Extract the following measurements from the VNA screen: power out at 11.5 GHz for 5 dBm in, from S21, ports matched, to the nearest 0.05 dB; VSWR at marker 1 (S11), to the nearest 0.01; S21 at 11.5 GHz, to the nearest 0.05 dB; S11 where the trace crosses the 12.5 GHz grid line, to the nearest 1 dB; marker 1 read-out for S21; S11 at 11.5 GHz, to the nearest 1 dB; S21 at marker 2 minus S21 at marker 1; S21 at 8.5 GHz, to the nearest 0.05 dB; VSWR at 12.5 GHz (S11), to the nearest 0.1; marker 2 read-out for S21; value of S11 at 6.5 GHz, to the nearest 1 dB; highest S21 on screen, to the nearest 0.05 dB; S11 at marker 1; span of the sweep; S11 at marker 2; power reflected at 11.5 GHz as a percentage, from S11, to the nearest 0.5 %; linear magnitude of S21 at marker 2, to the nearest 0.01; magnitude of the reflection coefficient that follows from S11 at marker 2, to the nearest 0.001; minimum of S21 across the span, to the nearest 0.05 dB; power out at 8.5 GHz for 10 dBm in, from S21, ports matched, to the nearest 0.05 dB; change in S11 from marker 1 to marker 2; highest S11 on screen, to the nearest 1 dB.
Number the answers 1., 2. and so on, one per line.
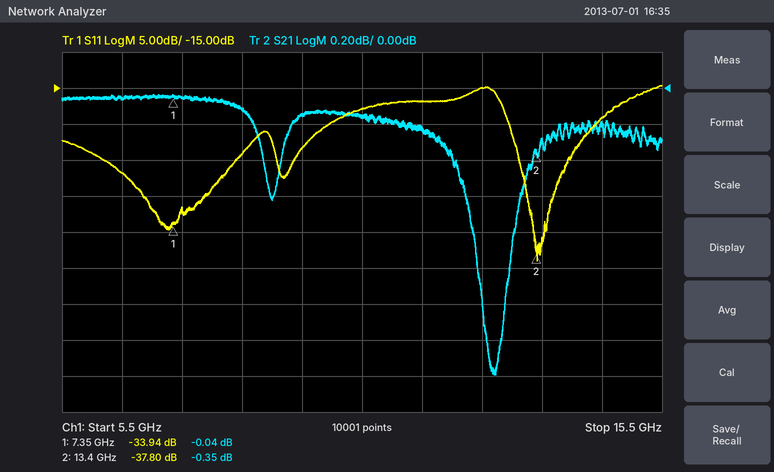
1. 4.75 dBm
2. 1.04
3. -0.25 dB
4. -15 dB
5. -0.04 dB
6. -17 dB
7. -0.31 dB
8. -0.10 dB
9. 1.4
10. -0.35 dB
11. -27 dB
12. -0.05 dB
13. -33.94 dB
14. 10 GHz
15. -37.80 dB
16. 2.0 %
17. 0.96
18. 0.013
19. -1.60 dB
20. 9.90 dBm
21. -3.86 dB
22. -15 dB
